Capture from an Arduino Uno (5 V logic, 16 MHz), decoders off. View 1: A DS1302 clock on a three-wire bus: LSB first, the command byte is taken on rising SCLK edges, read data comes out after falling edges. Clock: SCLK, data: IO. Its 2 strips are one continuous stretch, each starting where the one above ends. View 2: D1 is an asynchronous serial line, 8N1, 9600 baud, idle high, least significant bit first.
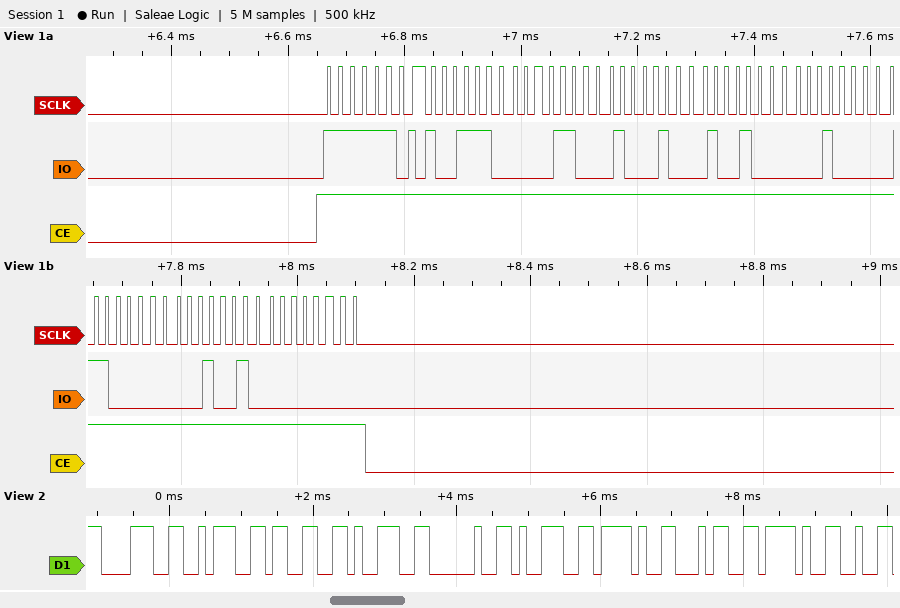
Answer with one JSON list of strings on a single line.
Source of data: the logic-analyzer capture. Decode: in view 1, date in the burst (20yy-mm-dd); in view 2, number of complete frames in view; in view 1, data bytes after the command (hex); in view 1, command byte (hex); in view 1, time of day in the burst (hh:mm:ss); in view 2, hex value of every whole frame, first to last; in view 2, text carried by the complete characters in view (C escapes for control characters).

["2024-04-09", "9", "39 18 11 09 04 03 24 00", "0xBF", "11:18:39", "0x38 0x3A 0x33 0x39 0x20 0x39 0x2F 0x34 0x2F", "\"8:39 9/4/\""]
